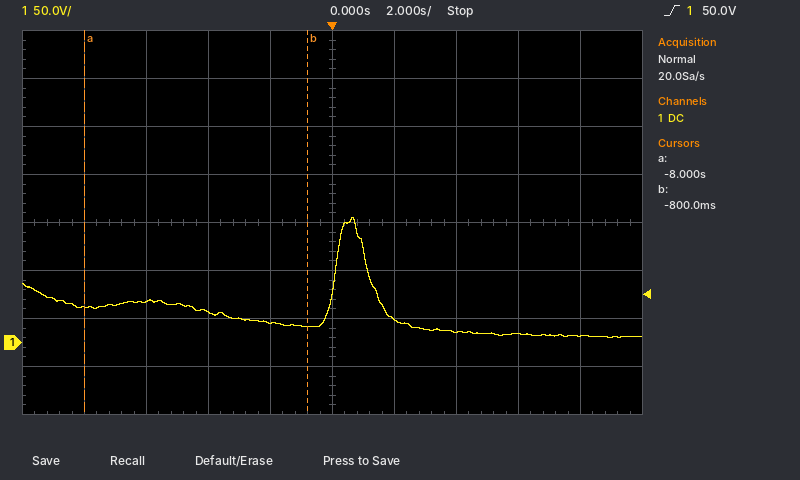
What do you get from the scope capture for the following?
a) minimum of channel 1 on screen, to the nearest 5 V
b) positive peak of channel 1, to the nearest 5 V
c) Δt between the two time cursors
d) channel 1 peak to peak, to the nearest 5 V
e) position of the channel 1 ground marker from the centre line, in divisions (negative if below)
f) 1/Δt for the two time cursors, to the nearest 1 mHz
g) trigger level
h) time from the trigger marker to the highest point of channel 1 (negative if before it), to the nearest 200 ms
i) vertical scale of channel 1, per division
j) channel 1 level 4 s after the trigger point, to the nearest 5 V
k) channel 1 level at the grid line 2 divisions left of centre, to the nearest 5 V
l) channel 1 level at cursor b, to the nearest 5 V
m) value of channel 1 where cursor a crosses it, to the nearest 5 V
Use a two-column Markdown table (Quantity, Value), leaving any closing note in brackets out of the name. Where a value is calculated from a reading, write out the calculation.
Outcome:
| Quantity | Value |
|---|---|
| minimum of channel 1 on screen, to the nearest 5 V | 5 V |
| positive peak of channel 1, to the nearest 5 V | 130 V |
| Δt between the two time cursors | -800 ms − (-8 s) = 7.2 s |
| channel 1 peak to peak, to the nearest 5 V | 130 V − (5 V) = 125 V |
| position of the channel 1 ground marker from the centre line, in divisions | -2.5 div |
| 1/Δt for the two time cursors, to the nearest 1 mHz | 1 / 7.2 s ≈ 139 mHz |
| trigger level | 50.0 V |
| time from the trigger marker to the highest point of channel 1 (negative if before it), to the nearest 200 ms | +600 ms |
| vertical scale of channel 1, per division | 50 V |
| channel 1 level 4 s after the trigger point, to the nearest 5 V | 10 V |
| channel 1 level at the grid line 2 divisions left of centre, to the nearest 5 V | 30 V |
| channel 1 level at cursor b, to the nearest 5 V | 15 V |
| value of channel 1 where cursor a crosses it, to the nearest 5 V | 35 V |
